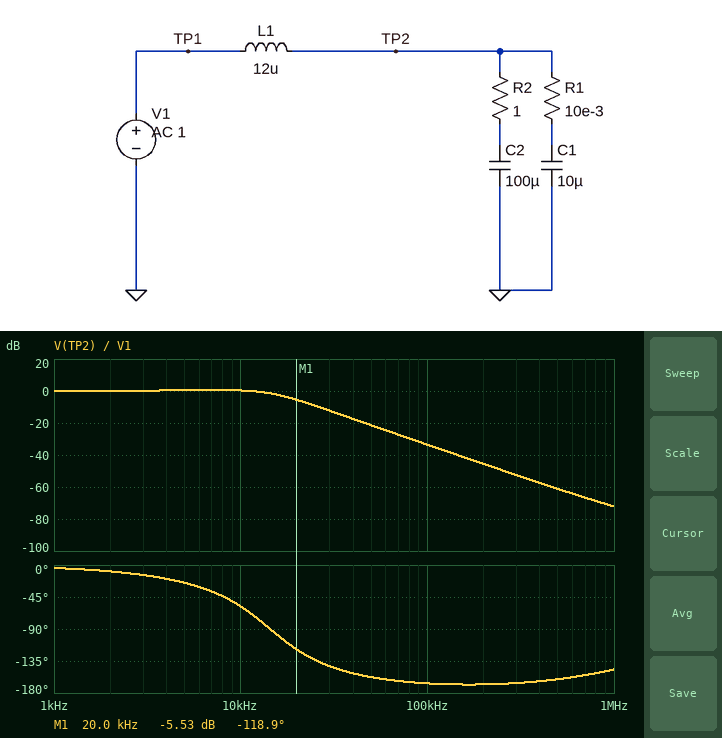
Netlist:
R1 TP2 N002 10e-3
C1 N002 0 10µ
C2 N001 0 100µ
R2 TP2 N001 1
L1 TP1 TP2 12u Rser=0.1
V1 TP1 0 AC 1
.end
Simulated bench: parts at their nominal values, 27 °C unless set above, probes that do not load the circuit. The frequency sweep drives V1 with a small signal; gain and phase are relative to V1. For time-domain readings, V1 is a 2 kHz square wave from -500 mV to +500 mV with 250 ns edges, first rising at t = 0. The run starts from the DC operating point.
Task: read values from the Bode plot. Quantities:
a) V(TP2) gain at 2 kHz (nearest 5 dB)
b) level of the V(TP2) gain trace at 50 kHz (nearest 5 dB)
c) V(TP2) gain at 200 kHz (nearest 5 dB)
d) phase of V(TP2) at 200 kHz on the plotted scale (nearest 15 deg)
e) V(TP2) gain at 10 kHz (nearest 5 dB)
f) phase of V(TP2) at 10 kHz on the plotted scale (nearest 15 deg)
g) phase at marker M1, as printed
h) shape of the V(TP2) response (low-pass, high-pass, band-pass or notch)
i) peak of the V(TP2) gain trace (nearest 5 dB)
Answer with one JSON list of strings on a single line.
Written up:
["0 dB", "-20 dB", "-45 dB", "-165 deg", "0 dB", "-60 deg", "-118.9 deg", "low-pass", "0 dB"]
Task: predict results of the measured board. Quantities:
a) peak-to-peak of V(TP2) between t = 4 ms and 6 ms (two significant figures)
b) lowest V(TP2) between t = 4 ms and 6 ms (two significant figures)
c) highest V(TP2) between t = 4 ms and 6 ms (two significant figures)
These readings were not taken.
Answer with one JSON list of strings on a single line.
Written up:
["1.2 V", "-610 mV", "610 mV"]
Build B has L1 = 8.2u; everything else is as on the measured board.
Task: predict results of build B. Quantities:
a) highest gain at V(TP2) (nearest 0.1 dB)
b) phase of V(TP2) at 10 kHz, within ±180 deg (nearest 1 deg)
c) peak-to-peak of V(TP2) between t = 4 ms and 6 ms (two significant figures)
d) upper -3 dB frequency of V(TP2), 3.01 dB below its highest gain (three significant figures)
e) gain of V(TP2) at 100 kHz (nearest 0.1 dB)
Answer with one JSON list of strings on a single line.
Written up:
["1.0 dB", "-40 deg", "1.3 V", "20.6 kHz", "-30.1 dB"]
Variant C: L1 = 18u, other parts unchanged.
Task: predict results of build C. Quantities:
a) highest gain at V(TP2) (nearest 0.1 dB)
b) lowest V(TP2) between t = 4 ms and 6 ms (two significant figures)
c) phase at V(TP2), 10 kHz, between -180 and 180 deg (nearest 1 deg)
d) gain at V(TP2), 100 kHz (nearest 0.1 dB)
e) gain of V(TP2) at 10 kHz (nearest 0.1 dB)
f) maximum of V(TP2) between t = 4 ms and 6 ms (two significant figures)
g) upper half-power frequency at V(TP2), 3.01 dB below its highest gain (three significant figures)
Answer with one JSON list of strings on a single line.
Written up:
["0.6 dB", "-600 mV", "-80 deg", "-37.1 dB", "-1.6 dB", "600 mV", "11.1 kHz"]
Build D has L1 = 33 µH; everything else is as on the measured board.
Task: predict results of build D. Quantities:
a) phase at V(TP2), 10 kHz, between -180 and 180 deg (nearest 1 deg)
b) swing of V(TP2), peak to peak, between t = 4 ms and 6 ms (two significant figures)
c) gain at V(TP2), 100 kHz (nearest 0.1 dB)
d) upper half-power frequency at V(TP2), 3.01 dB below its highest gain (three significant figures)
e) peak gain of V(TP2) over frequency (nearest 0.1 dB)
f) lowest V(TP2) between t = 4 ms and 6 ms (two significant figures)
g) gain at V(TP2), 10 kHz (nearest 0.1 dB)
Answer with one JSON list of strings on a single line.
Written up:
["-104 deg", "1.3 V", "-42.4 dB", "5.75 kHz", "1.3 dB", "-640 mV", "-6.7 dB"]
